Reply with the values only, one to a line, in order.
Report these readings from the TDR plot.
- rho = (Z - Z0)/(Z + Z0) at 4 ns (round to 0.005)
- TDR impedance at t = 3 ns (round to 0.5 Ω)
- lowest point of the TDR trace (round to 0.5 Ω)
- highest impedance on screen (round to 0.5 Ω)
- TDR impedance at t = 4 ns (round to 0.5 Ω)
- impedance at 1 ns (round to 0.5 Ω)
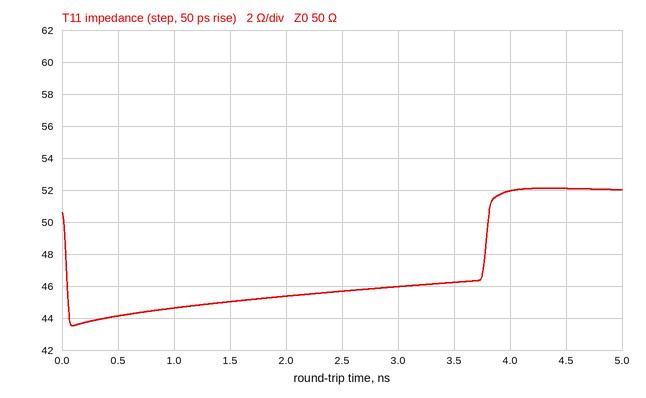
+0.020
46.0 Ω
43.5 Ω
52.0 Ω
52.0 Ω
44.5 Ω
